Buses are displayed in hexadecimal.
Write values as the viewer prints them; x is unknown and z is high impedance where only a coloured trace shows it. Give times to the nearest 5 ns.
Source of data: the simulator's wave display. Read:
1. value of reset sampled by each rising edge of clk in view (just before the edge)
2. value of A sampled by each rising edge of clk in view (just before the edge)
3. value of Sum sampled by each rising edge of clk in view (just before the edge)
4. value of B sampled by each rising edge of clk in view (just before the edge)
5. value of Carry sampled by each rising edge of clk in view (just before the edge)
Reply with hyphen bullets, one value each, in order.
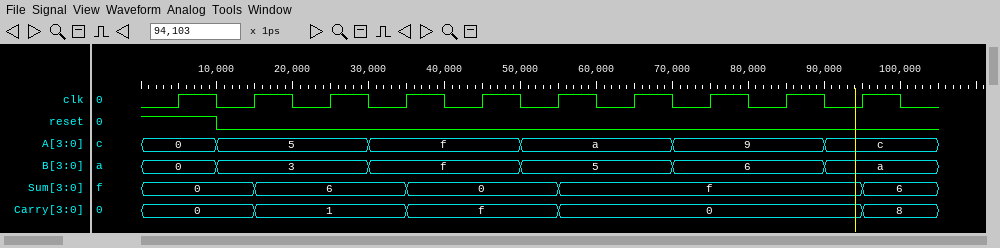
- 1 0 0 0 0 0 0 0 0 0
- 0, 5, 5, f, f, a, a, 9, 9, c
- 0, 0, 6, 6, 0, 0, f, f, f, f
- 0, 3, 3, f, f, 5, 5, 6, 6, a
- 0, 0, 1, 1, f, f, 0, 0, 0, 0
